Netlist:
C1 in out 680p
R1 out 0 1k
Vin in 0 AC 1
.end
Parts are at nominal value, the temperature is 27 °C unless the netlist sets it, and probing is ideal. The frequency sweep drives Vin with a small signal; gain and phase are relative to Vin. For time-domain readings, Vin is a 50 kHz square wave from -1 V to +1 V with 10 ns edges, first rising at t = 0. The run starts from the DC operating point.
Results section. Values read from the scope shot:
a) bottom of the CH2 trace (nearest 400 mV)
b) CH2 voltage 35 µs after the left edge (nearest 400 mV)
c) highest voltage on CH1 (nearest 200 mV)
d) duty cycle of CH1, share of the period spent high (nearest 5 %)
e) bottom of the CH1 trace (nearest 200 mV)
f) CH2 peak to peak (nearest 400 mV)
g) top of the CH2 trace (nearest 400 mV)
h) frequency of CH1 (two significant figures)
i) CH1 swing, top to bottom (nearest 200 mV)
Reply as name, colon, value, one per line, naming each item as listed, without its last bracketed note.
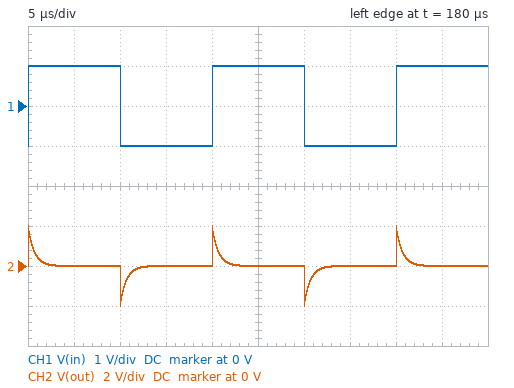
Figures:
bottom of the CH2 trace: -2.0 V
CH2 voltage 35 µs after the left edge: 0 V
highest voltage on CH1: 1.0 V
duty cycle of CH1, share of the period spent high: 50 %
bottom of the CH1 trace: -1.0 V
CH2 peak to peak: 4.0 V
top of the CH2 trace: 2.0 V
frequency of CH1: 50 kHz
CH1 swing, top to bottom: 2.0 V
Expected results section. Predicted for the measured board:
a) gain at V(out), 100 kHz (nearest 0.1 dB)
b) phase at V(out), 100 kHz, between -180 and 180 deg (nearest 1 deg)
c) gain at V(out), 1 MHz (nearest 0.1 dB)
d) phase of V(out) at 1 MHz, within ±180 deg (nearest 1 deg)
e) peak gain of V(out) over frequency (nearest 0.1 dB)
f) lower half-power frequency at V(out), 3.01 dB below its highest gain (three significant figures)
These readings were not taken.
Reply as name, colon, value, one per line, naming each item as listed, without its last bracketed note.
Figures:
gain at V(out), 100 kHz: -8.1 dB
phase at V(out), 100 kHz, between -180 and 180 deg: 67 deg
gain at V(out), 1 MHz: -0.2 dB
phase of V(out) at 1 MHz, within ±180 deg: 13 deg
peak gain of V(out) over frequency: 0 dB
lower half-power frequency at V(out), 3.01 dB below its highest gain: 234 kHz
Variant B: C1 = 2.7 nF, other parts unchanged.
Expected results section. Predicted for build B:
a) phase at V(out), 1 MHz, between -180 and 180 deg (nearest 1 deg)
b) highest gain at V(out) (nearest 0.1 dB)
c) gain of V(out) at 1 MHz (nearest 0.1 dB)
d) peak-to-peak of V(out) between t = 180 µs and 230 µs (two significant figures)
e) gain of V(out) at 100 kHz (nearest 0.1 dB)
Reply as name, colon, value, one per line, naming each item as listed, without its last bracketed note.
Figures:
phase at V(out), 1 MHz, between -180 and 180 deg: 3 deg
highest gain at V(out): 0 dB
gain of V(out) at 1 MHz: 0 dB
peak-to-peak of V(out) between t = 180 µs and 230 µs: 3.9 V
gain of V(out) at 100 kHz: -1.3 dB
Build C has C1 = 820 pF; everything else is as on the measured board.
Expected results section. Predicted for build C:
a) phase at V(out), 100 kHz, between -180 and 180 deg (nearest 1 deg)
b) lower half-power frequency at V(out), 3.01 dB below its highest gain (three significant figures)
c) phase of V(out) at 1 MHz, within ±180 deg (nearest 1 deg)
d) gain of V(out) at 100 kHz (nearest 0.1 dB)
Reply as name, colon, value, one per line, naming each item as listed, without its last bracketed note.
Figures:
phase at V(out), 100 kHz, between -180 and 180 deg: 63 deg
lower half-power frequency at V(out), 3.01 dB below its highest gain: 194 kHz
phase of V(out) at 1 MHz, within ±180 deg: 11 deg
gain of V(out) at 100 kHz: -6.8 dB
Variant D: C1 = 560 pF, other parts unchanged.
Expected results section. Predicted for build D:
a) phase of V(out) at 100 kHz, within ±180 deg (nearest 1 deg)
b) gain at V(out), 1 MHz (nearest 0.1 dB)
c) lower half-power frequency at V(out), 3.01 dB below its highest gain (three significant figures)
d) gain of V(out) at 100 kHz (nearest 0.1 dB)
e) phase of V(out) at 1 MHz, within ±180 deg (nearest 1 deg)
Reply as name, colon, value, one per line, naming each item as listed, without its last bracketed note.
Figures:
phase of V(out) at 100 kHz, within ±180 deg: 71 deg
gain at V(out), 1 MHz: -0.3 dB
lower half-power frequency at V(out), 3.01 dB below its highest gain: 284 kHz
gain of V(out) at 100 kHz: -9.6 dB
phase of V(out) at 1 MHz, within ±180 deg: 16 deg
